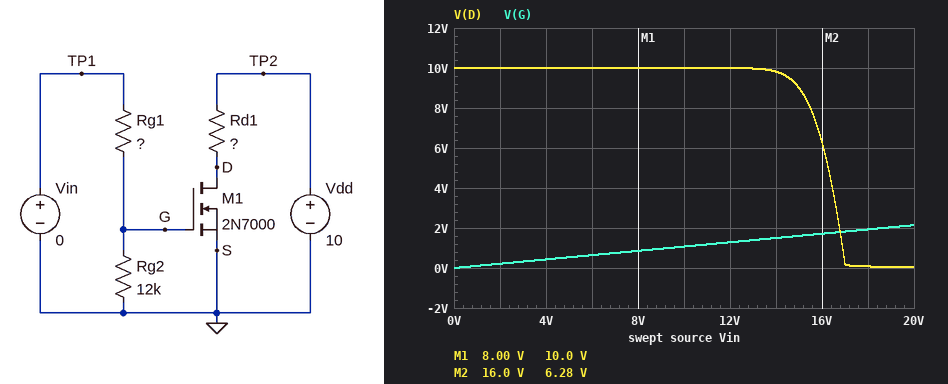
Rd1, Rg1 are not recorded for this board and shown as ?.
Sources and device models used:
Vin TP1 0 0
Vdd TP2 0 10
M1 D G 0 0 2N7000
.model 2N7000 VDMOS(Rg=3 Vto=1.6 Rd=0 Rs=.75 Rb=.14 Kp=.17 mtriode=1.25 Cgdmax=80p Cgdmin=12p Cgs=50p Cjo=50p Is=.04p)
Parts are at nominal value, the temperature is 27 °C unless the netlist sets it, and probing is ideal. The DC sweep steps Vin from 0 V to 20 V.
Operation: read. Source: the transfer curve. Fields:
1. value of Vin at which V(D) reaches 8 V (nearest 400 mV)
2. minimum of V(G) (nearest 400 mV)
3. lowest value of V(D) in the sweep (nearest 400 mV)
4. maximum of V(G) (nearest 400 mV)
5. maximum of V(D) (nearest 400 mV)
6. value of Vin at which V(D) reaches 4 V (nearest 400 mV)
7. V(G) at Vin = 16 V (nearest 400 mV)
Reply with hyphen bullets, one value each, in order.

- 15.6 V
- 0 V
- 0 V
- 2.0 V
- 10.0 V
- 16.4 V
- 1.6 V
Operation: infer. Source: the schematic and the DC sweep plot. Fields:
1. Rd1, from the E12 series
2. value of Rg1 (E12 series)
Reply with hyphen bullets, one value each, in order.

- 2.2 kΩ
- 100 kΩ
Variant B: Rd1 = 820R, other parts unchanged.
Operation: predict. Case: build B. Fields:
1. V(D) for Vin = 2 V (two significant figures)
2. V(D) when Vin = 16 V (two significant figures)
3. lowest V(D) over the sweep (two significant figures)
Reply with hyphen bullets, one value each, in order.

- 10 V
- 8.6 V
- 130 mV
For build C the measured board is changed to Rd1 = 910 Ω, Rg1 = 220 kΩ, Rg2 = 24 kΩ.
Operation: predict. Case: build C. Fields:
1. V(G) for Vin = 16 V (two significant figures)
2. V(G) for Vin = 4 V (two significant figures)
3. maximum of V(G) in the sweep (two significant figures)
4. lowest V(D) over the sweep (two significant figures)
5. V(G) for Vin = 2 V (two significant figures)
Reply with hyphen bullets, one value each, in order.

- 1.6 V
- 390 mV
- 2.0 V
- 240 mV
- 200 mV
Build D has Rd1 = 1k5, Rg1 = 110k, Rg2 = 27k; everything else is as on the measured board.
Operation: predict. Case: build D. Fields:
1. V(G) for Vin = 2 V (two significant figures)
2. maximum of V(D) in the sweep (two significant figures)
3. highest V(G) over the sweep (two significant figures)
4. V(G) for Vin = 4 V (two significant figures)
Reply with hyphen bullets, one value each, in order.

- 390 mV
- 10 V
- 3.9 V
- 790 mV
